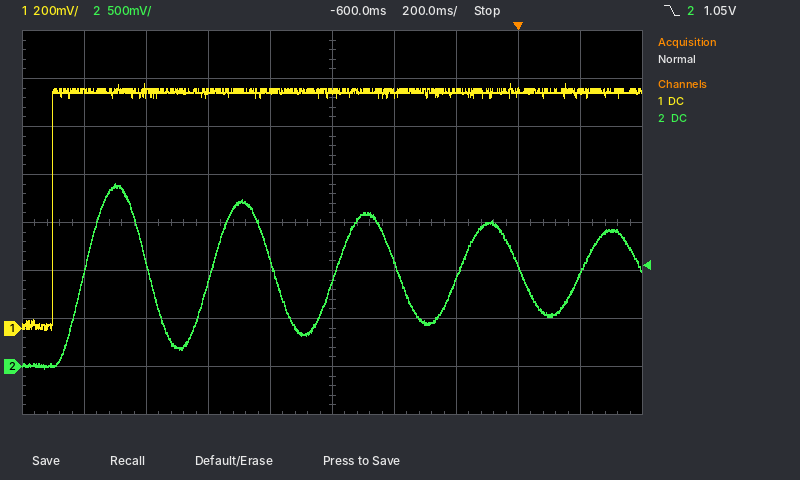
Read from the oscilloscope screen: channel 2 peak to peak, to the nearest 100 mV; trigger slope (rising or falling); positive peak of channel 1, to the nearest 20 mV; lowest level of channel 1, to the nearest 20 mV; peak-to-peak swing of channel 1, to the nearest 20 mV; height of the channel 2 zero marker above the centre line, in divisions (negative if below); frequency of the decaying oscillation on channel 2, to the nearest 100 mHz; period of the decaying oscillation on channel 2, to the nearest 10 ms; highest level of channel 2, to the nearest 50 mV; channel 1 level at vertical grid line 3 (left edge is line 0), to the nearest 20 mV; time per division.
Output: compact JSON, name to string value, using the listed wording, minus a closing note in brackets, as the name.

{"channel 2 peak to peak, to the nearest 100 mV": "1.90 V", "trigger slope": "falling", "positive peak of channel 1, to the nearest 20 mV": "1.02 V", "lowest level of channel 1, to the nearest 20 mV": "0 mV", "peak-to-peak swing of channel 1, to the nearest 20 mV": "1.02 V", "height of the channel 2 zero marker above the centre line, in divisions": "-3.0 div", "frequency of the decaying oscillation on channel 2, to the nearest 100 mHz": "2.5 Hz", "period of the decaying oscillation on channel 2, to the nearest 10 ms": "400 ms", "highest level of channel 2, to the nearest 50 mV": "1.90 V", "channel 1 level at vertical grid line 3 (left edge is line 0), to the nearest 20 mV": "980 mV", "time per division": "200 ms"}
